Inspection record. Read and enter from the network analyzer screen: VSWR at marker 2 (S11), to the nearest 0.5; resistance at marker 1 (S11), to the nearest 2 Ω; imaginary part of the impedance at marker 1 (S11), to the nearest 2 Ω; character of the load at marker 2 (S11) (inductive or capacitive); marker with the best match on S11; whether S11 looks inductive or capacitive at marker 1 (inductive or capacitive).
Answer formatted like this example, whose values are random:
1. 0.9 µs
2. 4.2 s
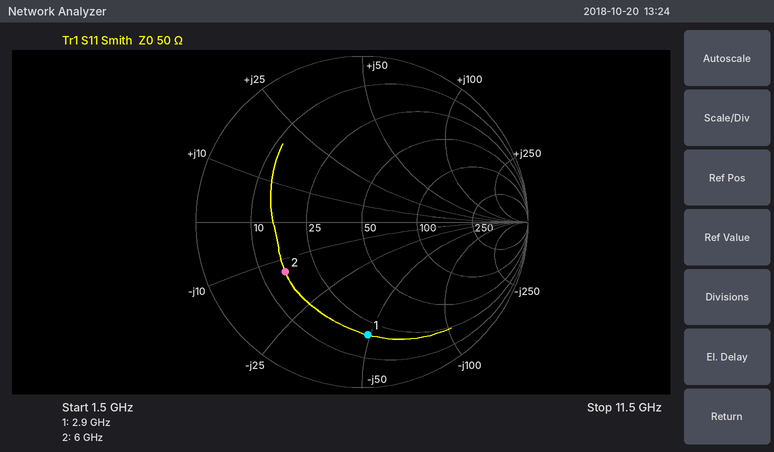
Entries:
1. 3.5
2. 20 Ω
3. -48 Ω
4. capacitive
5. marker 2
6. capacitive
